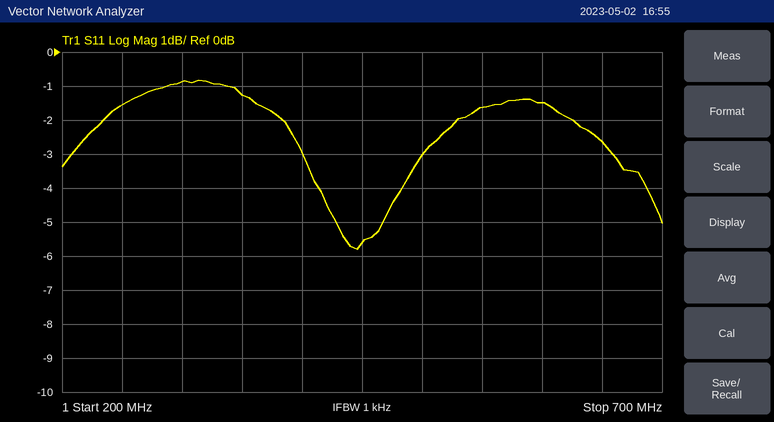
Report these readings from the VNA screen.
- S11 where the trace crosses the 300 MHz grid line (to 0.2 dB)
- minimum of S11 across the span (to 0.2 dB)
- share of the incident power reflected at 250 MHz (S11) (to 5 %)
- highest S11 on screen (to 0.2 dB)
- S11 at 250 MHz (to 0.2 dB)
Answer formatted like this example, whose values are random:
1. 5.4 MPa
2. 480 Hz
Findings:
1. -0.8 dB
2. -5.8 dB
3. 70 %
4. -0.8 dB
5. -1.6 dB
